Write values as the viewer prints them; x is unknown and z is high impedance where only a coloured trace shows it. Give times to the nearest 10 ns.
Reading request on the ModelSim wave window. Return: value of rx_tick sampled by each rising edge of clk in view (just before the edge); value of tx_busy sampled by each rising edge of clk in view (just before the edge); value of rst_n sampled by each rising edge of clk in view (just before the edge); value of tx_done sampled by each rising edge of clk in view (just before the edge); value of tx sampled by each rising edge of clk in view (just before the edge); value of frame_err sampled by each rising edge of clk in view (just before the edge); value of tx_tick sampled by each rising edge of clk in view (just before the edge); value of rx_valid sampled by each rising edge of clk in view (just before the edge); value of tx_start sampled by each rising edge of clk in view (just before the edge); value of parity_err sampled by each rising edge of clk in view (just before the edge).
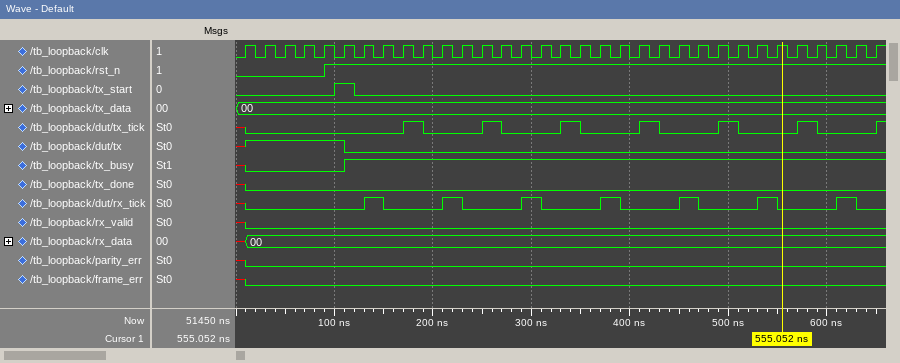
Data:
x 0 0 0 0 0 0 1 0 0 0 1 0 0 0 1 0 0 0 1 0 0 0 1 0 0 0 1 0 0 0 1 0
x 0 0 0 0 0 1 1 1 1 1 1 1 1 1 1 1 1 1 1 1 1 1 1 1 1 1 1 1 1 1 1 1
0 0 0 0 0 1 1 1 1 1 1 1 1 1 1 1 1 1 1 1 1 1 1 1 1 1 1 1 1 1 1 1 1
x 0 0 0 0 0 0 0 0 0 0 0 0 0 0 0 0 0 0 0 0 0 0 0 0 0 0 0 0 0 0 0 0
x 1 1 1 1 1 0 0 0 0 0 0 0 0 0 0 0 0 0 0 0 0 0 0 0 0 0 0 0 0 0 0 0
x 0 0 0 0 0 0 0 0 0 0 0 0 0 0 0 0 0 0 0 0 0 0 0 0 0 0 0 0 0 0 0 0
x 0 0 0 0 0 0 0 0 1 0 0 0 1 0 0 0 1 0 0 0 1 0 0 0 1 0 0 0 1 0 0 0
x 0 0 0 0 0 0 0 0 0 0 0 0 0 0 0 0 0 0 0 0 0 0 0 0 0 0 0 0 0 0 0 0
0 0 0 0 0 1 0 0 0 0 0 0 0 0 0 0 0 0 0 0 0 0 0 0 0 0 0 0 0 0 0 0 0
x 0 0 0 0 0 0 0 0 0 0 0 0 0 0 0 0 0 0 0 0 0 0 0 0 0 0 0 0 0 0 0 0
